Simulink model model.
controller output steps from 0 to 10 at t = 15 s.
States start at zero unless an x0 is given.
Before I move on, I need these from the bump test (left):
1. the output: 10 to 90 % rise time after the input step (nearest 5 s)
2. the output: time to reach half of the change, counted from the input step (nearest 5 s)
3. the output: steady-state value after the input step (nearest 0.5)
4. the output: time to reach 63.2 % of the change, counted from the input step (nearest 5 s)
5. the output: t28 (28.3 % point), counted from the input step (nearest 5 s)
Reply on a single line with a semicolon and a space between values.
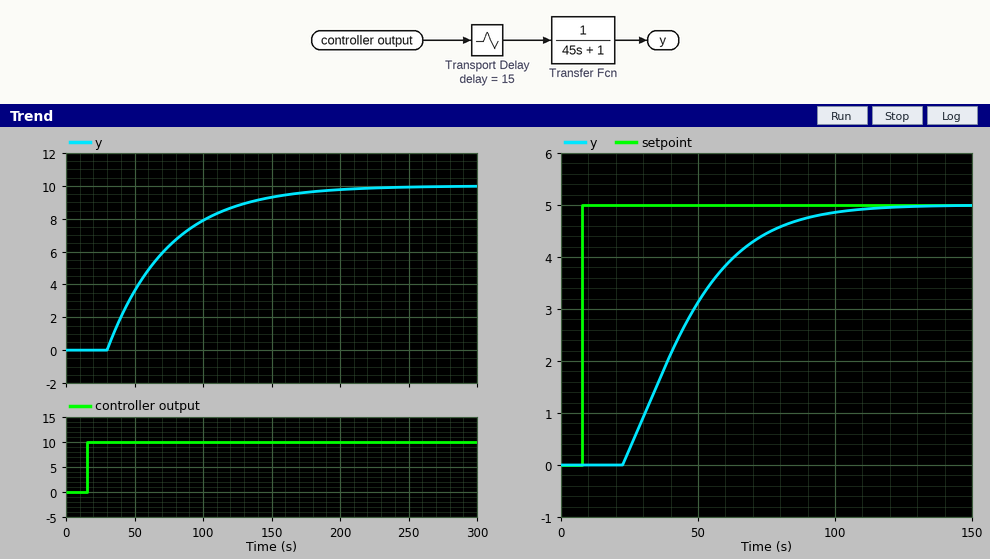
100 s; 45 s; 10.0; 60 s; 30 s
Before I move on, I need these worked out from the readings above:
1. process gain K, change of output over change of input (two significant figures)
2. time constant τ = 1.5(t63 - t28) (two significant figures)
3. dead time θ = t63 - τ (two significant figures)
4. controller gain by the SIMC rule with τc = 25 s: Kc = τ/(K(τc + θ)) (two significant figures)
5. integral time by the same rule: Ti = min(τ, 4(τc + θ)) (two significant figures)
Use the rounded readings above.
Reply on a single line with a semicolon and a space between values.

1.0; 45 s; 15 s; 1.1; 45 s
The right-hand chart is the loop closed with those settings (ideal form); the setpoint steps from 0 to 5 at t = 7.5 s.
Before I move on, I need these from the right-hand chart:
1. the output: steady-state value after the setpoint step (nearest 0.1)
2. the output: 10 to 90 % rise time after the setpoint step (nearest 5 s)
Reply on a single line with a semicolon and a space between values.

5.0; 50 s
